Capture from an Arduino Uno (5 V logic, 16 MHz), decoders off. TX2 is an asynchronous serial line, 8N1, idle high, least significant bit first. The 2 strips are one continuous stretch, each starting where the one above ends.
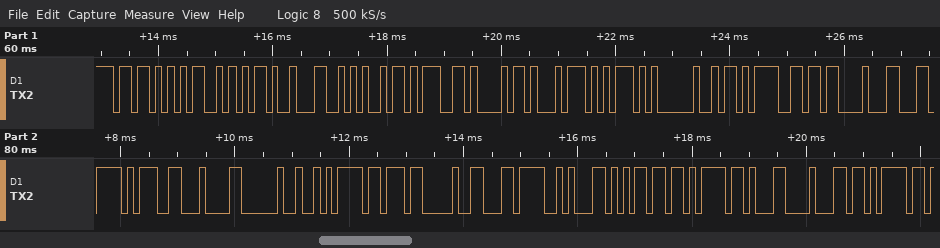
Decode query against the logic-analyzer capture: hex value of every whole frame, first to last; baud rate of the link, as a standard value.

5B 4D 2D 4C 69 67 68 74 5D 20 EB B6 88 EC 9D 84 20 EA BB 90 EC 8A B5 EB 8B 88 EB
9600 baud
